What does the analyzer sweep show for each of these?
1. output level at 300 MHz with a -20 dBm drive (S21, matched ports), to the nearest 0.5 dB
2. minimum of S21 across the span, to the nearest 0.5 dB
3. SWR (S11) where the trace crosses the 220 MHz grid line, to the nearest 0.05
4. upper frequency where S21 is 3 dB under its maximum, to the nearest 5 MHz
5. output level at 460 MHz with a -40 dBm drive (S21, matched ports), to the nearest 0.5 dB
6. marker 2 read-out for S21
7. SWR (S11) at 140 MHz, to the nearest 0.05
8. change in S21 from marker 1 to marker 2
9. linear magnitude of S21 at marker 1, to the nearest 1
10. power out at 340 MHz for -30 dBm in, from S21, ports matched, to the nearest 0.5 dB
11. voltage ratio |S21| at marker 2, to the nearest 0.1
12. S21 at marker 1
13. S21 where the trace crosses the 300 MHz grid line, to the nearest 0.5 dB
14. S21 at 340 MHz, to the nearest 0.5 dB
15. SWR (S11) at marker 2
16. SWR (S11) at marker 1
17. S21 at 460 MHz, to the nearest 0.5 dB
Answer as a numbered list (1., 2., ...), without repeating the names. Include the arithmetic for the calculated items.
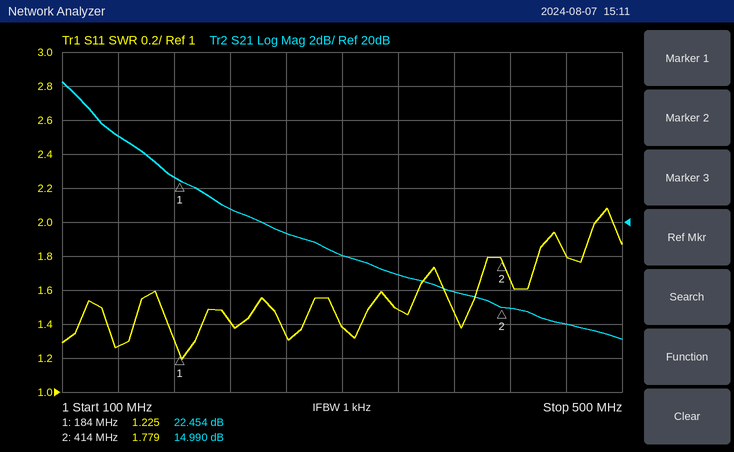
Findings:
1. -20 dBm + (18.0 dB) = -2.0 dBm
2. 13.0 dB
3. 1.40
4. 135 MHz
5. -40 dBm + (14.0 dB) = -26.0 dBm
6. 14.990 dB
7. 1.25
8. 14.99 − (22.454) = -7.464 dB
9. 10^(22.454/20) ≈ 13
10. -30 dBm + (17.0 dB) = -13.0 dBm
11. 10^(14.99/20) ≈ 5.6
12. 22.454 dB
13. 18.0 dB
14. 17.0 dB
15. 1.779
16. 1.225
17. 14.0 dB
